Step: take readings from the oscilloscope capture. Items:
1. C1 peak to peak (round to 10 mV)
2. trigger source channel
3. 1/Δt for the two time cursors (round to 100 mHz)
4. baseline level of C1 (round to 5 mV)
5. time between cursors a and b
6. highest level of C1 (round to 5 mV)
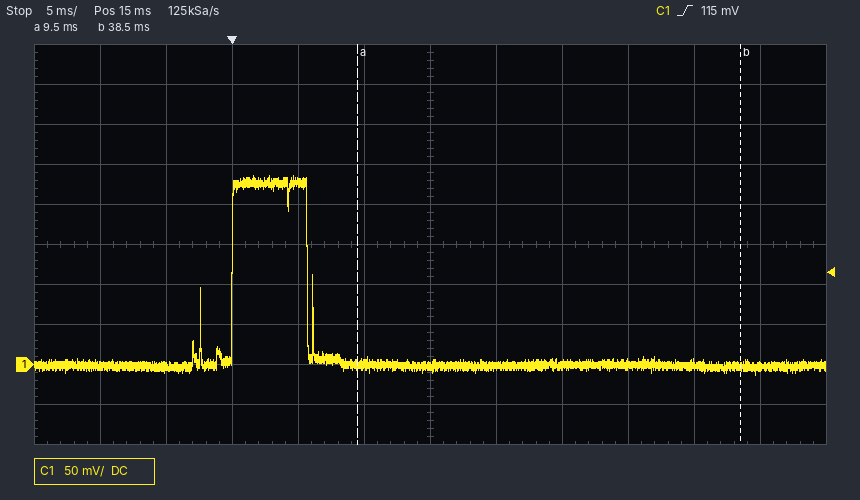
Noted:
250 mV
C1
34.5 Hz
0 mV
29.0 ms
235 mV
